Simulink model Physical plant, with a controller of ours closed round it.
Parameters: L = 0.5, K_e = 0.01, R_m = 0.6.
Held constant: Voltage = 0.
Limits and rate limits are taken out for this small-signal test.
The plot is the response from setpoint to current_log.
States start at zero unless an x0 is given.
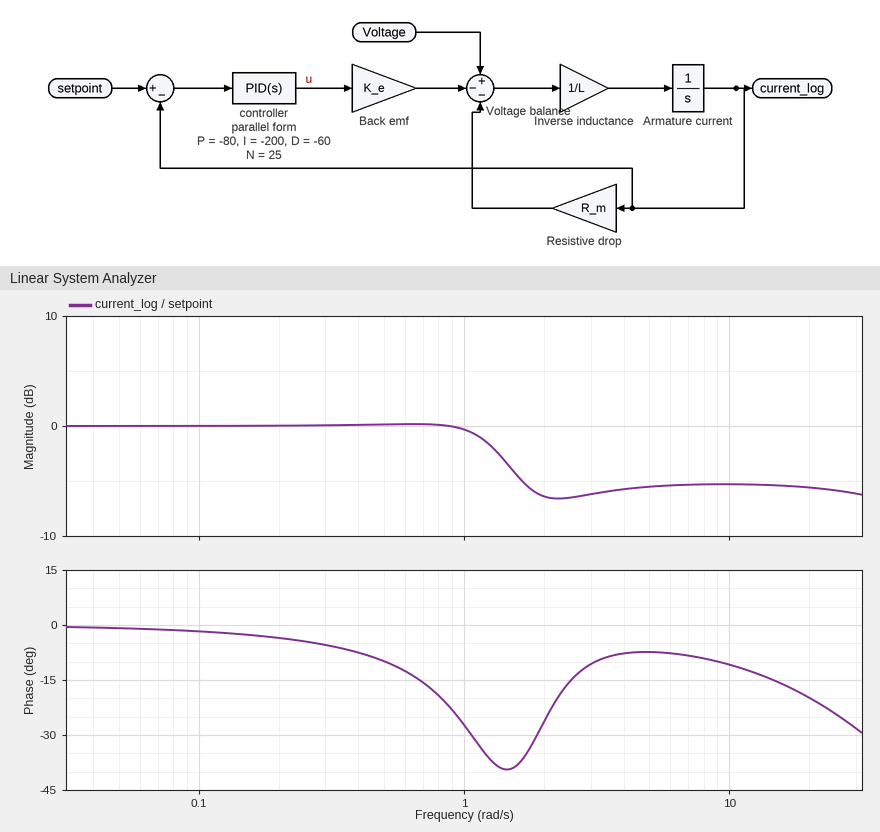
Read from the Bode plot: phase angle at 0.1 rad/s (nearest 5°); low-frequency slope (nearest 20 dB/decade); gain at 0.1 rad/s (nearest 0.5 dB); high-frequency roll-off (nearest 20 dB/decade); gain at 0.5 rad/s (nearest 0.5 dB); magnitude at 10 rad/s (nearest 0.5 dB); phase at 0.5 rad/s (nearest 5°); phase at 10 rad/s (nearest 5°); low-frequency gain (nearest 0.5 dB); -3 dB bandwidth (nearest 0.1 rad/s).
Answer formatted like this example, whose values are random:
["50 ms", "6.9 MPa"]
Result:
["0°", "0 dB/decade", "0.0 dB", "0 dB/decade", "0.0 dB", "-5.5 dB", "-10°", "-10°", "0.0 dB", "1.4 rad/s"]
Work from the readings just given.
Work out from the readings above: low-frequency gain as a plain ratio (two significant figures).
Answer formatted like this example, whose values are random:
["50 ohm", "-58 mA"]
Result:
["1.0"]
